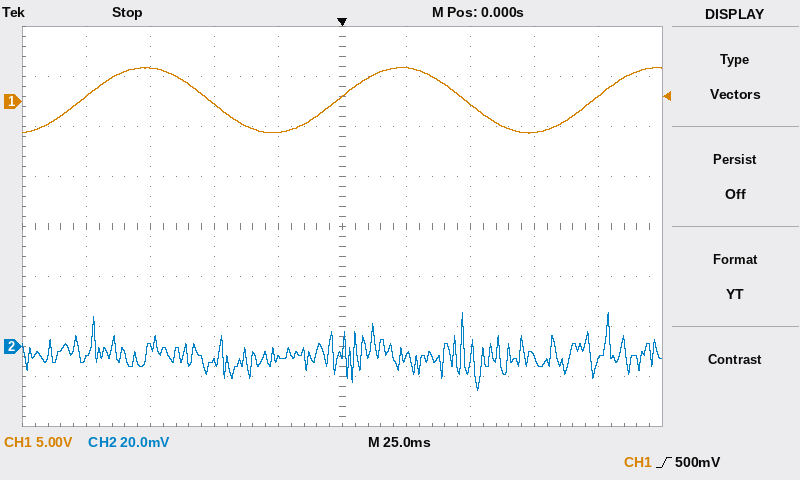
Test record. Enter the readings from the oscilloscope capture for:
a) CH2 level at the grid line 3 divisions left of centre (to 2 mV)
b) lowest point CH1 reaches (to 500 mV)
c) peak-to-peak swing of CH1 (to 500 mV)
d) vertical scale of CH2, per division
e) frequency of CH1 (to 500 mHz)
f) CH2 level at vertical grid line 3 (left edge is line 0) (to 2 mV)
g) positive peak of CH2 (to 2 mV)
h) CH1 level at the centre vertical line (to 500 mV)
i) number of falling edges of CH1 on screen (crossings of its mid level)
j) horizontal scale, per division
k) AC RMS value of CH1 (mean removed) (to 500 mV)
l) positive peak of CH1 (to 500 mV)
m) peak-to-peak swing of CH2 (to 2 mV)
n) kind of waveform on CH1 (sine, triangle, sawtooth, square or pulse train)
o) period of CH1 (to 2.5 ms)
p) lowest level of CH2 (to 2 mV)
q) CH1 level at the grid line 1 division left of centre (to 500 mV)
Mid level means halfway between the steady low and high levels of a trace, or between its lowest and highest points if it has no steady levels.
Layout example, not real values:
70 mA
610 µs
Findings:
0 mV
-3.0 V
6.5 V
20 mV
10.0 Hz
-6 mV
14 mV
500 mV
2
25 ms
2.5 V
3.5 V
32 mV
sine
100.0 ms
-18 mV
-3.0 V
